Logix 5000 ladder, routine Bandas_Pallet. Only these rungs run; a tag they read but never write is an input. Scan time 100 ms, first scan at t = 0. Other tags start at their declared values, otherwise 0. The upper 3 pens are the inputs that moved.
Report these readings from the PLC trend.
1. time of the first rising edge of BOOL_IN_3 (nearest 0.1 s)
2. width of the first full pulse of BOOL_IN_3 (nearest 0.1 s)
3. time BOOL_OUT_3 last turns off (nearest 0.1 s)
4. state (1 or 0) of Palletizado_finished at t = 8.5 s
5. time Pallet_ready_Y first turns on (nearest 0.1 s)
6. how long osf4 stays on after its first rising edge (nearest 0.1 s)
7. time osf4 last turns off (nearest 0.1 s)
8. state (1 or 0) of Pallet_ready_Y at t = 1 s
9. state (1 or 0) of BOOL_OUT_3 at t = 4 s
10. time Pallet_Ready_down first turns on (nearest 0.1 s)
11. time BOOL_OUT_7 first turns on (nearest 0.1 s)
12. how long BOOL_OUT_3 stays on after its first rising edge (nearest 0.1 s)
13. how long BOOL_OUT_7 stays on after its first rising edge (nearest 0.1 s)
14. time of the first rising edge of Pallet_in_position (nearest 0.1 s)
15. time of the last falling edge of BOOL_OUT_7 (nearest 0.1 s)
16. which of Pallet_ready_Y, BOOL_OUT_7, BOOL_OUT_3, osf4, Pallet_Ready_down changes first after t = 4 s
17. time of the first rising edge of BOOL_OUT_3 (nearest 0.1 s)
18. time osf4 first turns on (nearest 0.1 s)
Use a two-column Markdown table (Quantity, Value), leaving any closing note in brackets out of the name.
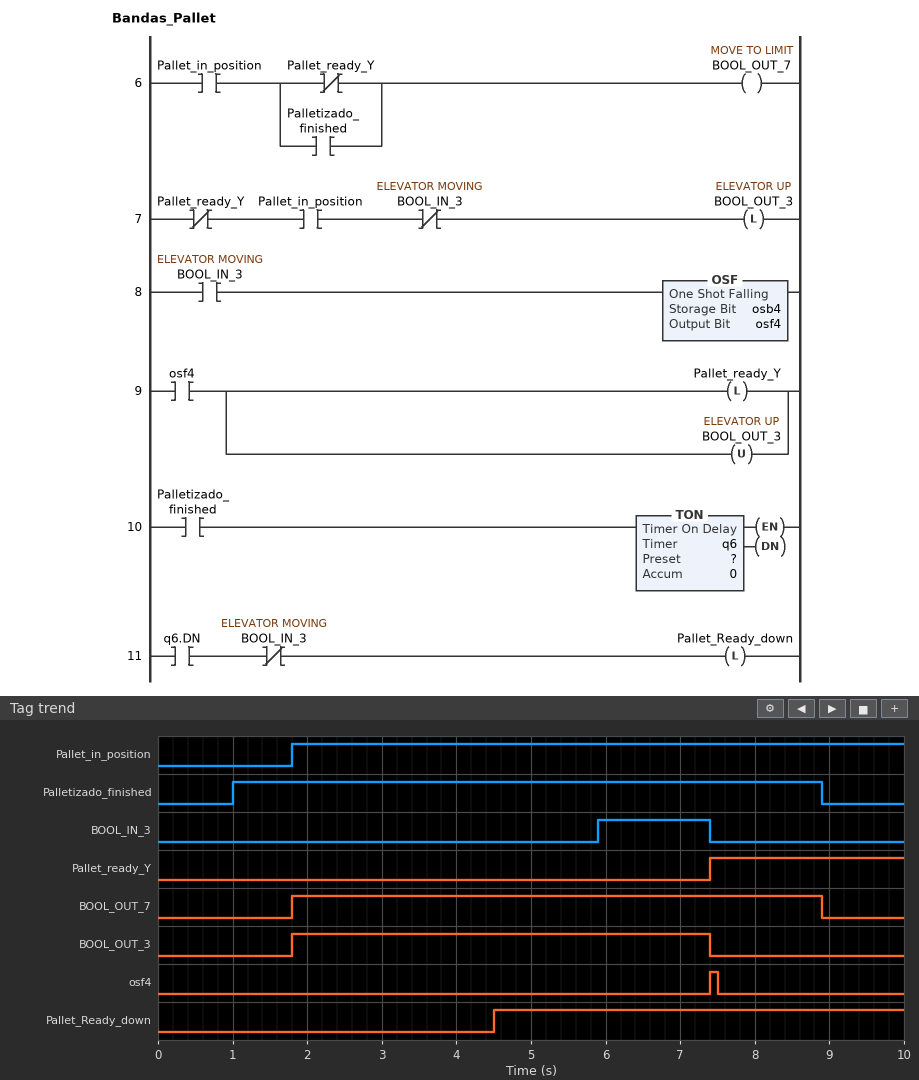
| Quantity | Value |
|---|---|
| time of the first rising edge of BOOL_IN_3 | 5.9 s |
| width of the first full pulse of BOOL_IN_3 | 1.5 s |
| time BOOL_OUT_3 last turns off | 7.4 s |
| state (1 or 0) of Palletizado_finished at t = 8.5 s | 1 |
| time Pallet_ready_Y first turns on | 7.4 s |
| how long osf4 stays on after its first rising edge | 0.1 s |
| time osf4 last turns off | 7.5 s |
| state (1 or 0) of Pallet_ready_Y at t = 1 s | 0 |
| state (1 or 0) of BOOL_OUT_3 at t = 4 s | 1 |
| time Pallet_Ready_down first turns on | 4.5 s |
| time BOOL_OUT_7 first turns on | 1.8 s |
| how long BOOL_OUT_3 stays on after its first rising edge | 5.6 s |
| how long BOOL_OUT_7 stays on after its first rising edge | 7.1 s |
| time of the first rising edge of Pallet_in_position | 1.8 s |
| time of the last falling edge of BOOL_OUT_7 | 8.9 s |
| which of Pallet_ready_Y, BOOL_OUT_7, BOOL_OUT_3, osf4, Pallet_Ready_down changes first after t = 4 s | Pallet_Ready_down |
| time of the first rising edge of BOOL_OUT_3 | 1.8 s |
| time osf4 first turns on | 7.4 s |
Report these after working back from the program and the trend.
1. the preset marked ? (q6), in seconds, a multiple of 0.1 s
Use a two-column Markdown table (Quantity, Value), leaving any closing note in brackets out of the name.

| Quantity | Value |
|---|---|
| the preset marked ? (q6), in seconds, a multiple of 0.1 s | 3.5 s |
